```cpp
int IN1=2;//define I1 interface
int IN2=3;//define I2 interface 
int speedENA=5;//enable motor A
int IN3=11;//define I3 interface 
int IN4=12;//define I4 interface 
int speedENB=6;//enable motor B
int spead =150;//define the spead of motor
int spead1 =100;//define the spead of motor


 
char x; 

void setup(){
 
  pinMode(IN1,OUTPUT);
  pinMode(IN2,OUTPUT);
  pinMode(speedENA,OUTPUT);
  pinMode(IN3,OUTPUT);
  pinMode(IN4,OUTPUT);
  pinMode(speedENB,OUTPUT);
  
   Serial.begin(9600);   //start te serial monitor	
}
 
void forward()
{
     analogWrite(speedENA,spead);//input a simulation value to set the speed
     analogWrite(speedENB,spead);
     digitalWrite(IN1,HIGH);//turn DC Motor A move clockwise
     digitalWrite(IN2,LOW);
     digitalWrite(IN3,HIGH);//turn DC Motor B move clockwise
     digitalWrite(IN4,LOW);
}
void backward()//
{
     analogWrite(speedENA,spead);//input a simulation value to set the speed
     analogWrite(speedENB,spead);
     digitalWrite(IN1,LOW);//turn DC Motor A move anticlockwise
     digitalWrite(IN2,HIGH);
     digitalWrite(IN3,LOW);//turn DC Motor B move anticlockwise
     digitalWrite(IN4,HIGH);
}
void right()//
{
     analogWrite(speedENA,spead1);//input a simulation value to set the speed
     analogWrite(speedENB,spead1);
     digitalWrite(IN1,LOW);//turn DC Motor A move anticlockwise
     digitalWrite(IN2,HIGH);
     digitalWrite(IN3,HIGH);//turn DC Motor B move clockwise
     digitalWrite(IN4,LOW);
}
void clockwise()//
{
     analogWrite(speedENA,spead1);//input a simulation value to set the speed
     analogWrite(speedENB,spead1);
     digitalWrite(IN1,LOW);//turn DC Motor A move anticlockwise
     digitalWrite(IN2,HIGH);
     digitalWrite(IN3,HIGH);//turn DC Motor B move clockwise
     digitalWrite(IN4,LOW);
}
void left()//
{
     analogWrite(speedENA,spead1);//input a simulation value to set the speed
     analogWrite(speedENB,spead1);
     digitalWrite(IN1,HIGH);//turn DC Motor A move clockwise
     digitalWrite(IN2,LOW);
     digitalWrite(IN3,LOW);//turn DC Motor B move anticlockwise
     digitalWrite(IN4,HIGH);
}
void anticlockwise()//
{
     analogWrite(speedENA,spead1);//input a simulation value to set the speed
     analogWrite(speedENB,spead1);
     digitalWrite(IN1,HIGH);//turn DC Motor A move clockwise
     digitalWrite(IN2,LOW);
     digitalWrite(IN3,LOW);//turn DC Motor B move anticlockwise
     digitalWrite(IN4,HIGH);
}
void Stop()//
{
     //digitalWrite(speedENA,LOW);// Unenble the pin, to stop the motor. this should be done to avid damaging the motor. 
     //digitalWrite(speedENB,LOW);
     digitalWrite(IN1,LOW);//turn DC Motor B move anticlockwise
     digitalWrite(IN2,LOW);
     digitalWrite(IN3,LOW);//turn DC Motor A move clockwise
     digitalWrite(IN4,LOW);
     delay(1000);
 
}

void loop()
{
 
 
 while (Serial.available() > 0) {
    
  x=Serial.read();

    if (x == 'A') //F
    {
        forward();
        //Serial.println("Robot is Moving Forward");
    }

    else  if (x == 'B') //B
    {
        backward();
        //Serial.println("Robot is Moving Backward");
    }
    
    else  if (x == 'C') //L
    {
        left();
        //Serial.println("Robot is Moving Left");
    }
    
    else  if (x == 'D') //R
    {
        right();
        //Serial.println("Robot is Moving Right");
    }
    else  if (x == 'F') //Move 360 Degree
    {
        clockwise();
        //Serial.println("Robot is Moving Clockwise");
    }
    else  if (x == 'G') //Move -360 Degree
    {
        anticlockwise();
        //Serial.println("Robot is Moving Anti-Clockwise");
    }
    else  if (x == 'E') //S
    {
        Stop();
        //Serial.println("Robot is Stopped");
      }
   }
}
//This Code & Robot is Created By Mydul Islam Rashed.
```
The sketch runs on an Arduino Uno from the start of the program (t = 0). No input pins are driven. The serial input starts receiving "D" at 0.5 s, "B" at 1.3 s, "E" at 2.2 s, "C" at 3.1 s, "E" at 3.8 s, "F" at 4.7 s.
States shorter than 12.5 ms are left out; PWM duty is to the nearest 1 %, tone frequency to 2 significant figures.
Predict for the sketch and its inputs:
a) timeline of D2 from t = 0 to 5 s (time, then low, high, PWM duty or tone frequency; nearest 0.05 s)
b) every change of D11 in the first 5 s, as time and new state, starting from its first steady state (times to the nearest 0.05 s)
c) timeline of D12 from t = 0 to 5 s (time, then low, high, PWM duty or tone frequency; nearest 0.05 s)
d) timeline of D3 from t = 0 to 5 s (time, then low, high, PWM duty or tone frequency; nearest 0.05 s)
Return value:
0 s low; 3.2 s high; 3.8 s low
0 s low; 0.5 s high; 1.3 s low; 4.8 s high
0 s low; 1.3 s high; 2.2 s low; 3.2 s high; 3.8 s low
0 s low; 0.5 s high; 2.2 s low; 4.8 s high
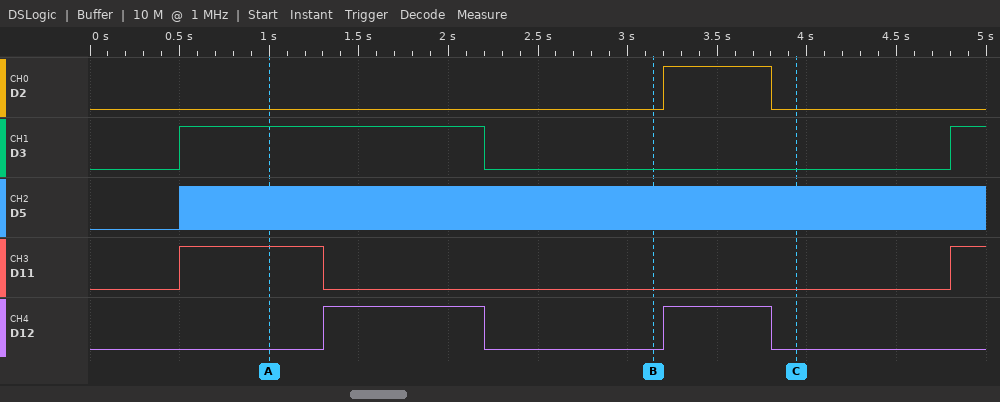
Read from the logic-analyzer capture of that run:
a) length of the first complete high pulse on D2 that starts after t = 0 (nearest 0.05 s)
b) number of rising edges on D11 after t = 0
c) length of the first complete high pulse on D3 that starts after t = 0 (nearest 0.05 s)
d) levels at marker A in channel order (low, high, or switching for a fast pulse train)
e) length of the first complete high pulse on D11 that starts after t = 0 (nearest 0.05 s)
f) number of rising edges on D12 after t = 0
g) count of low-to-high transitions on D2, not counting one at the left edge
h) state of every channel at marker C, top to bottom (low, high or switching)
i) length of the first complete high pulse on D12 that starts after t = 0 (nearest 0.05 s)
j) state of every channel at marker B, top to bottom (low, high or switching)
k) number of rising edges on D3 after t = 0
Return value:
0.60 s
2
1.70 s
D2 low, D3 high, D5 switching, D11 high, D12 low
0.80 s
2
1
D2 low, D3 low, D5 switching, D11 low, D12 low
0.90 s
D2 low, D3 low, D5 switching, D11 low, D12 low
2
